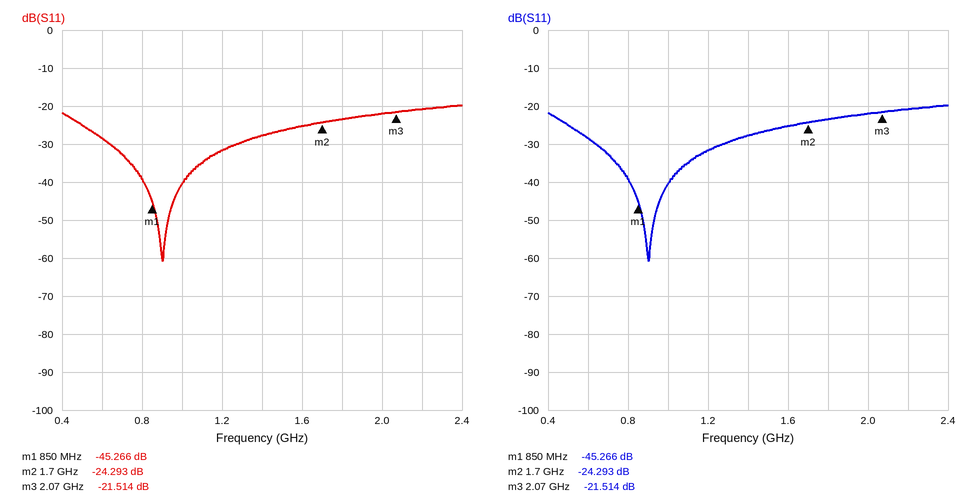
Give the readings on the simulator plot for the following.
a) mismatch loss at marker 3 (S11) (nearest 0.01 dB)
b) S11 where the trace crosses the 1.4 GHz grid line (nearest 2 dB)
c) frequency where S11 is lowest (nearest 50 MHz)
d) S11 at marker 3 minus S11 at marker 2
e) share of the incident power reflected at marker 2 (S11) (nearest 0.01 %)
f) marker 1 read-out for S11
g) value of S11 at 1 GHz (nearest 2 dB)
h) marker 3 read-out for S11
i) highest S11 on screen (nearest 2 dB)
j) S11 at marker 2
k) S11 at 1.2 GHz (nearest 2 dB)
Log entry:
0.03 dB
-28 dB
900 MHz
2.779 dB
0.37 %
-45.266 dB
-40 dB
-21.514 dB
-20 dB
-24.293 dB
-32 dB
